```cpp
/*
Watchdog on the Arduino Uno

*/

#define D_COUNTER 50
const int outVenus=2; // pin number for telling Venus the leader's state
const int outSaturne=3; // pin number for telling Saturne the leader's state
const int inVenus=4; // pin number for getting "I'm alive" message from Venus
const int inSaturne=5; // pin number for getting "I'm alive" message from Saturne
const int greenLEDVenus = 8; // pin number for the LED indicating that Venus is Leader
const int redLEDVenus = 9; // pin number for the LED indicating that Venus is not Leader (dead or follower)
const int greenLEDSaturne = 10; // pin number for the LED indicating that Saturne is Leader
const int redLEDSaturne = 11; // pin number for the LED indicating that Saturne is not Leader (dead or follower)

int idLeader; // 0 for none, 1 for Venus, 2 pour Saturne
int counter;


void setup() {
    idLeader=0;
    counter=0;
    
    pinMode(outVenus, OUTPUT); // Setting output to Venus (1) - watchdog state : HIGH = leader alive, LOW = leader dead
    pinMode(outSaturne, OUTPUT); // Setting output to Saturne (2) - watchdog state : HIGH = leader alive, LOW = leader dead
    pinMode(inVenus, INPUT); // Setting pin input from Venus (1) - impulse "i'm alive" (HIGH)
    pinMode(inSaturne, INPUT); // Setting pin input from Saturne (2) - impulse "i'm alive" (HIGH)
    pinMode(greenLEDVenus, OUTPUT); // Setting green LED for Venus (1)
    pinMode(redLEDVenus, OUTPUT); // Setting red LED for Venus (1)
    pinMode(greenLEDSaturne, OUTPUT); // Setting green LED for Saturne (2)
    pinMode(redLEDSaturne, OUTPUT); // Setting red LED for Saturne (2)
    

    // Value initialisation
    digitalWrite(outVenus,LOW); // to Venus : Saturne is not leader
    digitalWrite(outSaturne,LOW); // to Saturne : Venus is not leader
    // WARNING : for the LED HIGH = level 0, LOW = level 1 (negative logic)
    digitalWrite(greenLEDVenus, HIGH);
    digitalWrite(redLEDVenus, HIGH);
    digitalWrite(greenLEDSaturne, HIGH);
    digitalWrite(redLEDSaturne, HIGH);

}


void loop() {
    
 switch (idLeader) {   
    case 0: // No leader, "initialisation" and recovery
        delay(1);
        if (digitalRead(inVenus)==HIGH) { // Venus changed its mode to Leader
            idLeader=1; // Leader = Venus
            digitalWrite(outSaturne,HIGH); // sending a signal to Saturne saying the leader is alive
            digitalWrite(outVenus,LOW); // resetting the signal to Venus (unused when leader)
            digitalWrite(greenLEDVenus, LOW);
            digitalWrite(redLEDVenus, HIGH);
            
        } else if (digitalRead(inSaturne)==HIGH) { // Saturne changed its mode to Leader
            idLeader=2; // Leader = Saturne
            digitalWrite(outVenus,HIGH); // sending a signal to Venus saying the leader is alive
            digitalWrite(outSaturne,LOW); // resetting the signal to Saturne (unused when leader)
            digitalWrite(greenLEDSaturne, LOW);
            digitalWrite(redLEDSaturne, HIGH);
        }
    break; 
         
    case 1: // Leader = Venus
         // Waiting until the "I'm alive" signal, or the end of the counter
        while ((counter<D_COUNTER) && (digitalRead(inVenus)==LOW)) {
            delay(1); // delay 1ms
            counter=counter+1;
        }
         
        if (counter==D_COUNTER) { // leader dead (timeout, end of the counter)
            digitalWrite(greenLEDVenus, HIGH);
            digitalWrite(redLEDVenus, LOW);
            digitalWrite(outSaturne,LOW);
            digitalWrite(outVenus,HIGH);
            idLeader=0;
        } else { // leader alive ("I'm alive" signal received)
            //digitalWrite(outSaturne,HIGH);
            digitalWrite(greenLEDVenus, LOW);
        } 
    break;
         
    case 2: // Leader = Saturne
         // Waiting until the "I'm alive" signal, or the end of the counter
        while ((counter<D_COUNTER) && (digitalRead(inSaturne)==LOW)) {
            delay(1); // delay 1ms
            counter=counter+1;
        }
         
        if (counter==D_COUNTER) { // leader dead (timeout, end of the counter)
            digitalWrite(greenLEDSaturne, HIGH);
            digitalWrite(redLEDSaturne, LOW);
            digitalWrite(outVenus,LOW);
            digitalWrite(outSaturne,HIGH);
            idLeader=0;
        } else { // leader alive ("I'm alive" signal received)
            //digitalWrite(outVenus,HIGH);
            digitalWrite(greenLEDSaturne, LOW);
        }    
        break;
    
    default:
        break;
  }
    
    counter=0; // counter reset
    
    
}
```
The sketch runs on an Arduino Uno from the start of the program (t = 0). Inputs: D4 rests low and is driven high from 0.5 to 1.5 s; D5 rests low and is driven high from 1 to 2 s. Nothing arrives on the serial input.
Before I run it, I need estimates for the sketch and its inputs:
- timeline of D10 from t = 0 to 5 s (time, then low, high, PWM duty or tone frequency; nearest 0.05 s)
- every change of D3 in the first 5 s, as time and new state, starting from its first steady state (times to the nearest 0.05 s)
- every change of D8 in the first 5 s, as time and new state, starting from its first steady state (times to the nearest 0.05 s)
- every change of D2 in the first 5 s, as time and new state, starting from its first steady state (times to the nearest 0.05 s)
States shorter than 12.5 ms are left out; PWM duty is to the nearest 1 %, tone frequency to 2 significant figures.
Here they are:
0 s high; 1.55 s low; 2.05 s high
0 s low; 0.5 s high; 1.55 s low; 2.05 s high
0 s high; 0.5 s low; 1.55 s high
0 s low; 1.55 s high; 2.05 s low
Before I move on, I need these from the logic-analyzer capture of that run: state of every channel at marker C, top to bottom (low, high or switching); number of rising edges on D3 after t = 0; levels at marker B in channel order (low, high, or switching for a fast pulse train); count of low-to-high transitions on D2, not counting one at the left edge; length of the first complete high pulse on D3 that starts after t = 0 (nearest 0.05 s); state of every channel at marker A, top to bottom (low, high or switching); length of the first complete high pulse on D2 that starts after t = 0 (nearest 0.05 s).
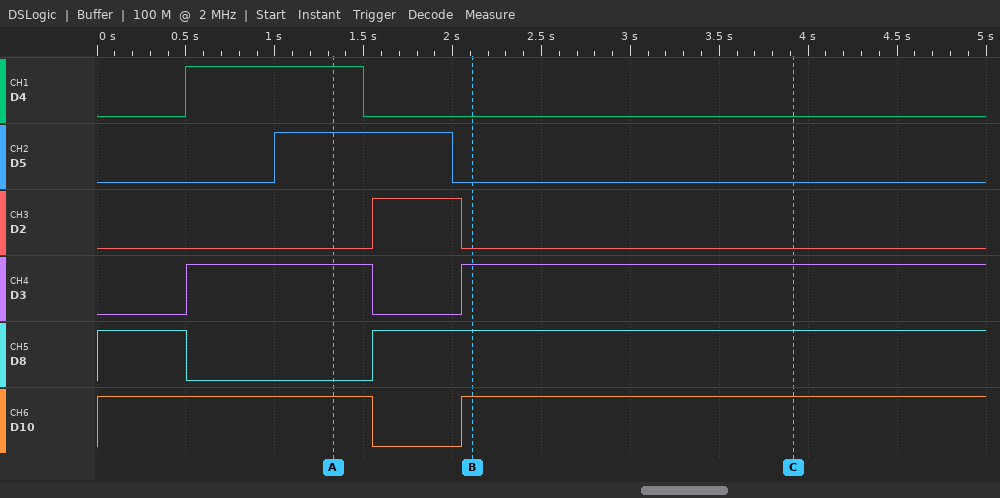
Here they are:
D4 low, D5 low, D2 low, D3 high, D8 high, D10 high
2
D4 low, D5 low, D2 low, D3 high, D8 high, D10 high
1
1.05 s
D4 high, D5 high, D2 low, D3 high, D8 low, D10 high
0.50 s
